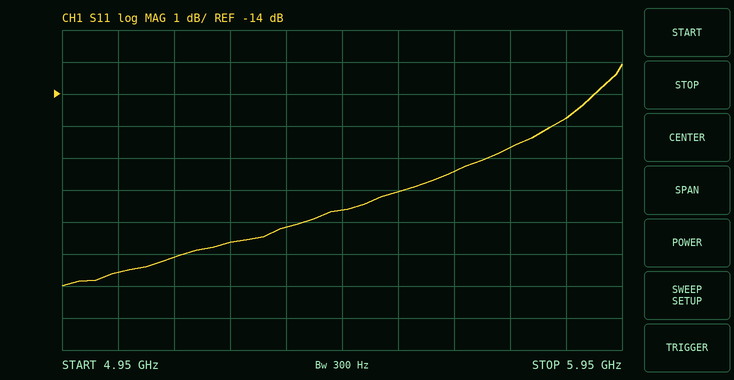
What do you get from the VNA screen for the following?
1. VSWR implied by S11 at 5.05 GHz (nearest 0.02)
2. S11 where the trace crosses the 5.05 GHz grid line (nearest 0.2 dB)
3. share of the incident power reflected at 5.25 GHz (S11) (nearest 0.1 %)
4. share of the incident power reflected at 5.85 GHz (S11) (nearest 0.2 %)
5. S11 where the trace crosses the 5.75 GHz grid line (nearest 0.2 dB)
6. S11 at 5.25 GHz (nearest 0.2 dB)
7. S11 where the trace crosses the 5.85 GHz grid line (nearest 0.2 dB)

1.24
-19.6 dB
1.4 %
3.4 %
-15.6 dB
-18.6 dB
-14.8 dB
